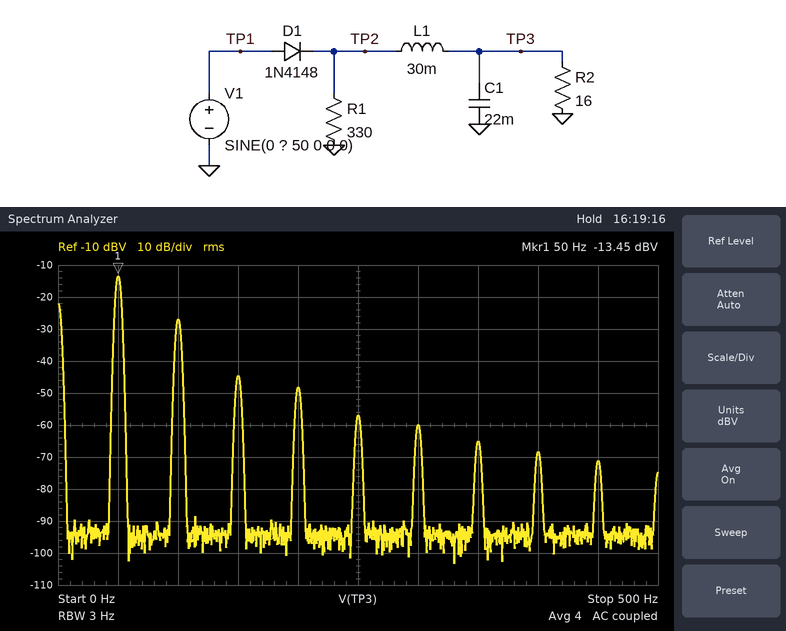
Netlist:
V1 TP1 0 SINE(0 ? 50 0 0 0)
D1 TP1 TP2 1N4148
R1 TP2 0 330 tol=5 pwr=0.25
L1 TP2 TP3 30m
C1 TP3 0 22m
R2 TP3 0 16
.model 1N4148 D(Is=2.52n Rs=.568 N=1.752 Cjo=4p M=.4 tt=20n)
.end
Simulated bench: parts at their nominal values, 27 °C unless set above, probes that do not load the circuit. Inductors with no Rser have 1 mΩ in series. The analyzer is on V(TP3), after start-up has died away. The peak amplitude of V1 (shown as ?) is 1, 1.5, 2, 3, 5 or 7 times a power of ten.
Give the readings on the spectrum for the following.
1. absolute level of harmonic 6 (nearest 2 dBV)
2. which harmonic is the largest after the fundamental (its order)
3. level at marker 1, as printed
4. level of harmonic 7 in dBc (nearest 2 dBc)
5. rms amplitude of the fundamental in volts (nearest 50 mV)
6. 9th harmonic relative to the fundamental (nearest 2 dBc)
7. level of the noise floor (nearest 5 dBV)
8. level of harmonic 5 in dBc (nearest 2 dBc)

-60 dBV
2
-13.45 dBV
-52 dBc
200 mV
-58 dBc
-95 dBV
-44 dBc
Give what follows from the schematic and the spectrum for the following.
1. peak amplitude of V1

50 V
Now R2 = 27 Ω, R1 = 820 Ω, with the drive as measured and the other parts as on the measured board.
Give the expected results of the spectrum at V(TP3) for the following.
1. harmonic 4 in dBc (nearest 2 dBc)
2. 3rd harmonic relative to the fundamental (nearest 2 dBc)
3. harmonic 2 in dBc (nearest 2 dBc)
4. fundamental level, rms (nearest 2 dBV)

-34 dBc
-28 dBc
-12 dBc
-16 dBV
